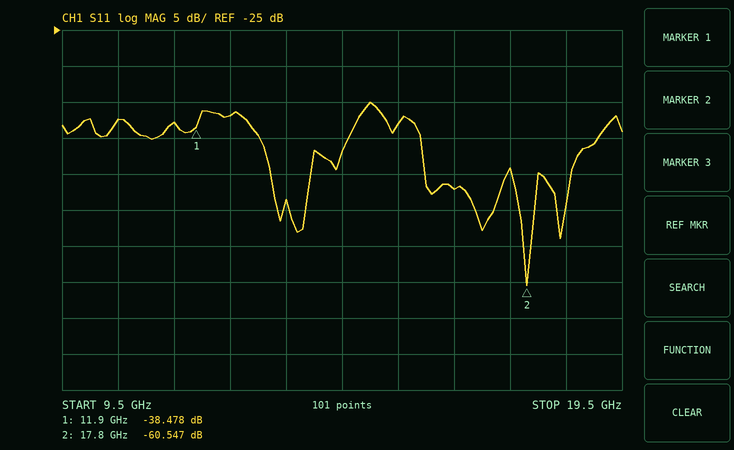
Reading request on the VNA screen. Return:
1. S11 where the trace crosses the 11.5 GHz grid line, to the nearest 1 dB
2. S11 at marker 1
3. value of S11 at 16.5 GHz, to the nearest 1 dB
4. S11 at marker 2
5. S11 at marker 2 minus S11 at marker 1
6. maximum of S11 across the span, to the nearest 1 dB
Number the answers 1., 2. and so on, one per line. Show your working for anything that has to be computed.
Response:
1. -38 dB
2. -38.478 dB
3. -47 dB
4. -60.547 dB
5. -60.547 − (-38.478) = -22.069 dB
6. -35 dB
